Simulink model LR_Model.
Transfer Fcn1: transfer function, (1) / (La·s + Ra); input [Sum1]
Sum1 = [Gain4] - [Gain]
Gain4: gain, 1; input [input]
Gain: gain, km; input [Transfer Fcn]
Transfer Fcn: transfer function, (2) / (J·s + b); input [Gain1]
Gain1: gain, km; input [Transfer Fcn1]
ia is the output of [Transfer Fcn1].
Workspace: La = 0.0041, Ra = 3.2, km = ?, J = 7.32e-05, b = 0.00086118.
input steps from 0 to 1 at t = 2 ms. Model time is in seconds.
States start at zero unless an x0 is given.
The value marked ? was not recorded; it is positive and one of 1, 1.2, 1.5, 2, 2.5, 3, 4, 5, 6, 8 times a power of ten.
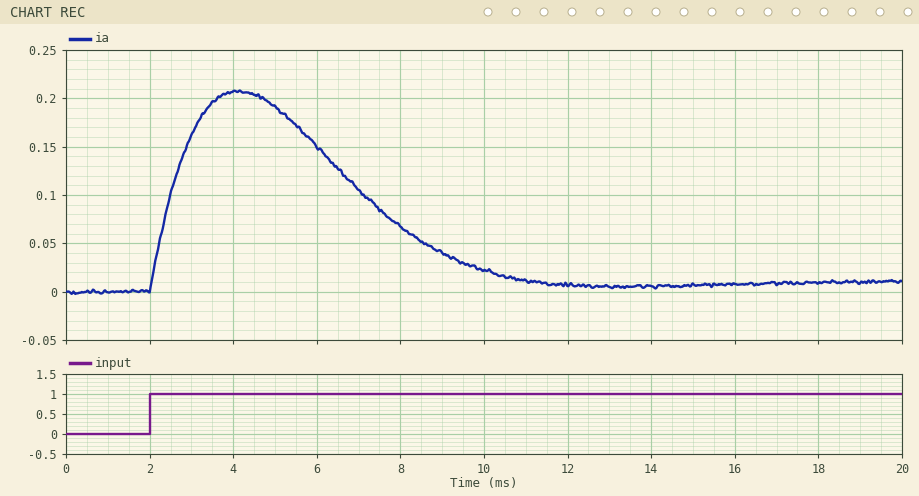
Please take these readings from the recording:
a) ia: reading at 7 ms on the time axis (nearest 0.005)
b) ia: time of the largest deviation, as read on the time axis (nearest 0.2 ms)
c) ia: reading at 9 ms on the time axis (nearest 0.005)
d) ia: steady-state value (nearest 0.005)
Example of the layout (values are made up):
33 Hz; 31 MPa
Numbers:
0.105; 4.2 ms; 0.040; 0.010
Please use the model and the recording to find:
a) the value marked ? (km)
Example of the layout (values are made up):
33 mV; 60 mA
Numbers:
0.2
